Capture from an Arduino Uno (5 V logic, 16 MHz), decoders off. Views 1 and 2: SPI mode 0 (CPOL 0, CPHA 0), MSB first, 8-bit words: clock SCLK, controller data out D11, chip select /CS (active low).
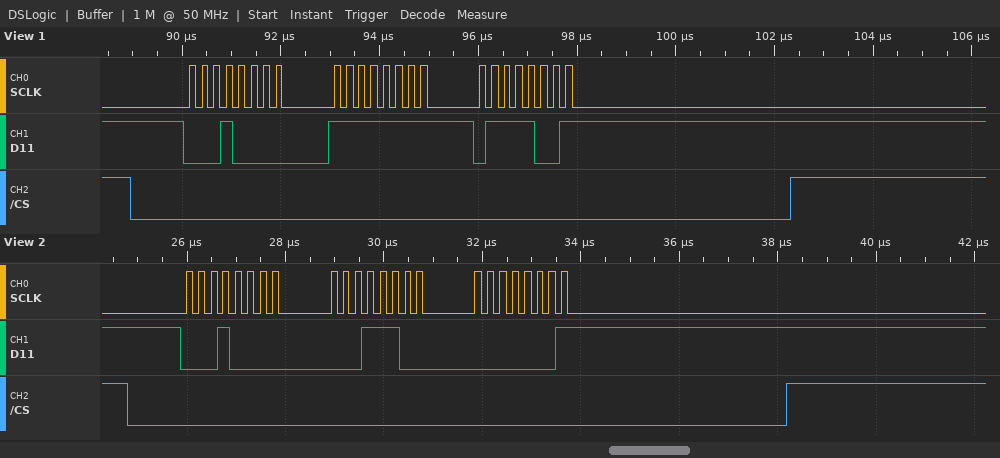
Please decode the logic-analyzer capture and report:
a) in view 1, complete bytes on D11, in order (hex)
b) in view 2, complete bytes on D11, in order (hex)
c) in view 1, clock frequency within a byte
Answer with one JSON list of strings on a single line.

["10 FF 79", "10 1C 01", "4 MHz"]
